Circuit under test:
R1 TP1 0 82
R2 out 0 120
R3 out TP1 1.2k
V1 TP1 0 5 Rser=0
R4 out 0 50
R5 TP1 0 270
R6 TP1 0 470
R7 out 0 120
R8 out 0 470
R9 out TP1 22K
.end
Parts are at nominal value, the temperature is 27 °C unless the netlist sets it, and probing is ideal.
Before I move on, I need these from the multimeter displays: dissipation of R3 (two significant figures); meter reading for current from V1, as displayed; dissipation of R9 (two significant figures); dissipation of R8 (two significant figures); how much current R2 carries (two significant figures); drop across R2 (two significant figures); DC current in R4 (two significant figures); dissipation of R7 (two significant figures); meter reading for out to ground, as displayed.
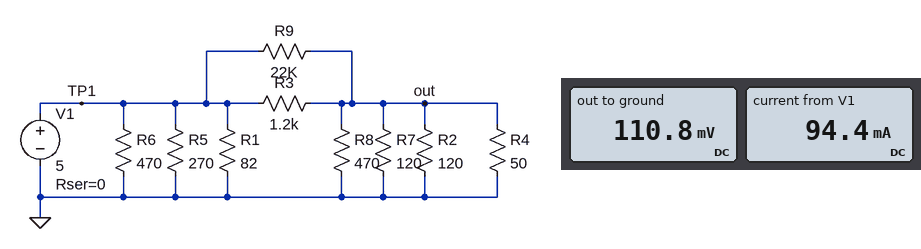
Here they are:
20 mW
94.4 mA
1.1 mW
26 µW
920 µA
110 mV
2.2 mA
100 µW
110.8 mV
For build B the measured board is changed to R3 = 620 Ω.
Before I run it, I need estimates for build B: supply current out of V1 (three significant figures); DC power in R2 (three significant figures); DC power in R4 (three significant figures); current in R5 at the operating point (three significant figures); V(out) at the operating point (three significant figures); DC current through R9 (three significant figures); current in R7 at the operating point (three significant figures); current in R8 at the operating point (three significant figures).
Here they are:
98.1 mA
350 µW
840 µW
18.5 mA
205 mV
218 µA
1.71 mA
436 µA
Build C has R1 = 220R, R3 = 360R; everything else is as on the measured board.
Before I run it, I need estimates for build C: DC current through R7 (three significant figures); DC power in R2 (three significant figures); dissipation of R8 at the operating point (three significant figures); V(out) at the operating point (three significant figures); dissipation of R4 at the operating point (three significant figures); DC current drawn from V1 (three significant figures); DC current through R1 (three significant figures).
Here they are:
2.83 mA
959 µW
245 µW
339 mV
2.30 mW
65.0 mA
22.7 mA
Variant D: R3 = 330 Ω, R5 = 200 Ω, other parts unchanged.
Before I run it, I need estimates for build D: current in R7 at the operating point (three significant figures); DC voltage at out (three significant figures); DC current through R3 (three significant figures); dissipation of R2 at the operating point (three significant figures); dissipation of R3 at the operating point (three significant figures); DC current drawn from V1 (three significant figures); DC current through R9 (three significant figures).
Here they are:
3.06 mA
367 mV
14.0 mA
1.12 mW
65.0 mW
111 mA
211 µA
